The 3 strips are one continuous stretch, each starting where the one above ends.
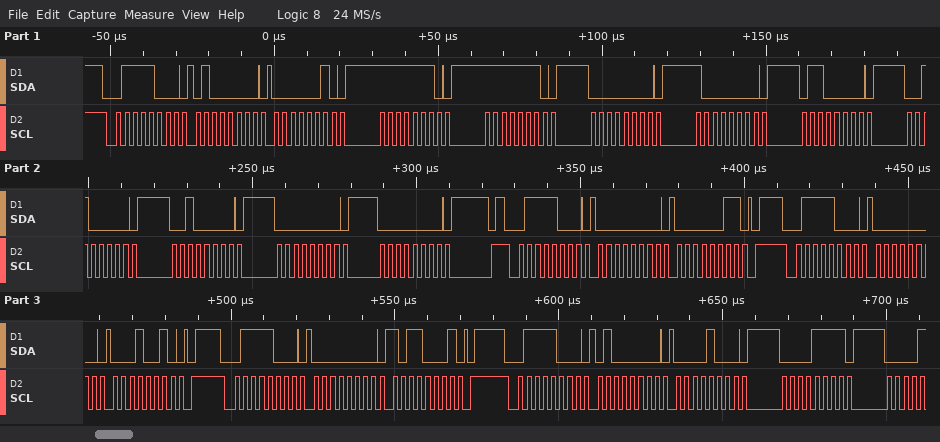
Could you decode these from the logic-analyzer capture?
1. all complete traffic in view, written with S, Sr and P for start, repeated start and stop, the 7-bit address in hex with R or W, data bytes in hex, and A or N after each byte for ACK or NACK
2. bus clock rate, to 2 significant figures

S 3CW A 40 A 02 A FE A FE A 00 A 80 A 60 A 20 A 20 A 00 A 00 A P S 3CW A 00 A 03 A P S 3CW A 00 A 12 A P S 3CW A 00 A B1 A P S 3CW A 40 A 08 A 0F A
400 kHz
